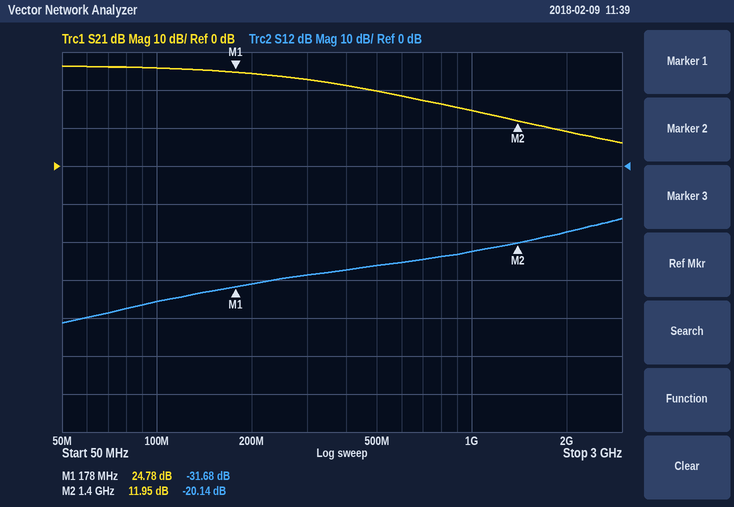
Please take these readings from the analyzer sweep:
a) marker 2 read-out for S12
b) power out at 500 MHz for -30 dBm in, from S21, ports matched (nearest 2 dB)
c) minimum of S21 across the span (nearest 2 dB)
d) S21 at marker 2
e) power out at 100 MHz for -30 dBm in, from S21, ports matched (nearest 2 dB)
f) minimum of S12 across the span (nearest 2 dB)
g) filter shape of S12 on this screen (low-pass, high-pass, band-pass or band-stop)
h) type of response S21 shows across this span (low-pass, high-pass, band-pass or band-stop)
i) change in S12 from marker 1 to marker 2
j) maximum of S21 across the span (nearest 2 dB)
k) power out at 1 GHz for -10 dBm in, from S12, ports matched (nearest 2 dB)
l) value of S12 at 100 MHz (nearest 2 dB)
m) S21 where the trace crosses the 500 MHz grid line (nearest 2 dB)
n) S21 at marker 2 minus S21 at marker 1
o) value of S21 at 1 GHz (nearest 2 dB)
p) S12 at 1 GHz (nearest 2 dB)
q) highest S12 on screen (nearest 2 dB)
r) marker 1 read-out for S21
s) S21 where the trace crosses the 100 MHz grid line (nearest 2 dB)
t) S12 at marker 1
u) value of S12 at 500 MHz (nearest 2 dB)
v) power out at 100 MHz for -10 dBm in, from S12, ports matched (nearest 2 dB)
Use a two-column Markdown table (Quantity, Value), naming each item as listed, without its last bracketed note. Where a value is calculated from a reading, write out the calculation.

| Quantity | Value |
|---|---|
| marker 2 read-out for S12 | -20.14 dB |
| power out at 500 MHz for -30 dBm in, from S21, ports matched | -30 dBm + (20 dB) = -10 dBm |
| minimum of S21 across the span | 6 dB |
| S21 at marker 2 | 11.95 dB |
| power out at 100 MHz for -30 dBm in, from S21, ports matched | -30 dBm + (26 dB) = -4 dBm |
| minimum of S12 across the span | -42 dB |
| filter shape of S12 on this screen | high-pass |
| type of response S21 shows across this span | low-pass |
| change in S12 from marker 1 to marker 2 | -20.14 − (-31.68) = 11.54 dB |
| maximum of S21 across the span | 26 dB |
| power out at 1 GHz for -10 dBm in, from S12, ports matched | -10 dBm + (-22 dB) = -32 dBm |
| value of S12 at 100 MHz | -36 dB |
| S21 where the trace crosses the 500 MHz grid line | 20 dB |
| S21 at marker 2 minus S21 at marker 1 | 11.95 − (24.78) = -12.83 dB |
| value of S21 at 1 GHz | 14 dB |
| S12 at 1 GHz | -22 dB |
| highest S12 on screen | -14 dB |
| marker 1 read-out for S21 | 24.78 dB |
| S21 where the trace crosses the 100 MHz grid line | 26 dB |
| S12 at marker 1 | -31.68 dB |
| value of S12 at 500 MHz | -26 dB |
| power out at 100 MHz for -10 dBm in, from S12, ports matched | -10 dBm + (-36 dB) = -46 dBm |
